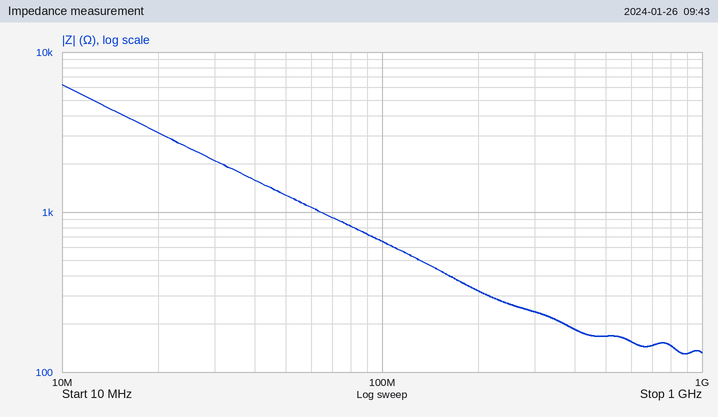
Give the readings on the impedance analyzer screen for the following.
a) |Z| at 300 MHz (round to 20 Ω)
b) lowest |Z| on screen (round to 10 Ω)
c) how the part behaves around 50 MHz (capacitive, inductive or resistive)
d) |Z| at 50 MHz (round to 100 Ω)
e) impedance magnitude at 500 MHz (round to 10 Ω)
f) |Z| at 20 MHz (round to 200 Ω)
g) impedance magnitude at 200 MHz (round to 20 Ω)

240 Ω
130 Ω
capacitive
1.3 kΩ
170 Ω
3.2 kΩ
320 Ω
